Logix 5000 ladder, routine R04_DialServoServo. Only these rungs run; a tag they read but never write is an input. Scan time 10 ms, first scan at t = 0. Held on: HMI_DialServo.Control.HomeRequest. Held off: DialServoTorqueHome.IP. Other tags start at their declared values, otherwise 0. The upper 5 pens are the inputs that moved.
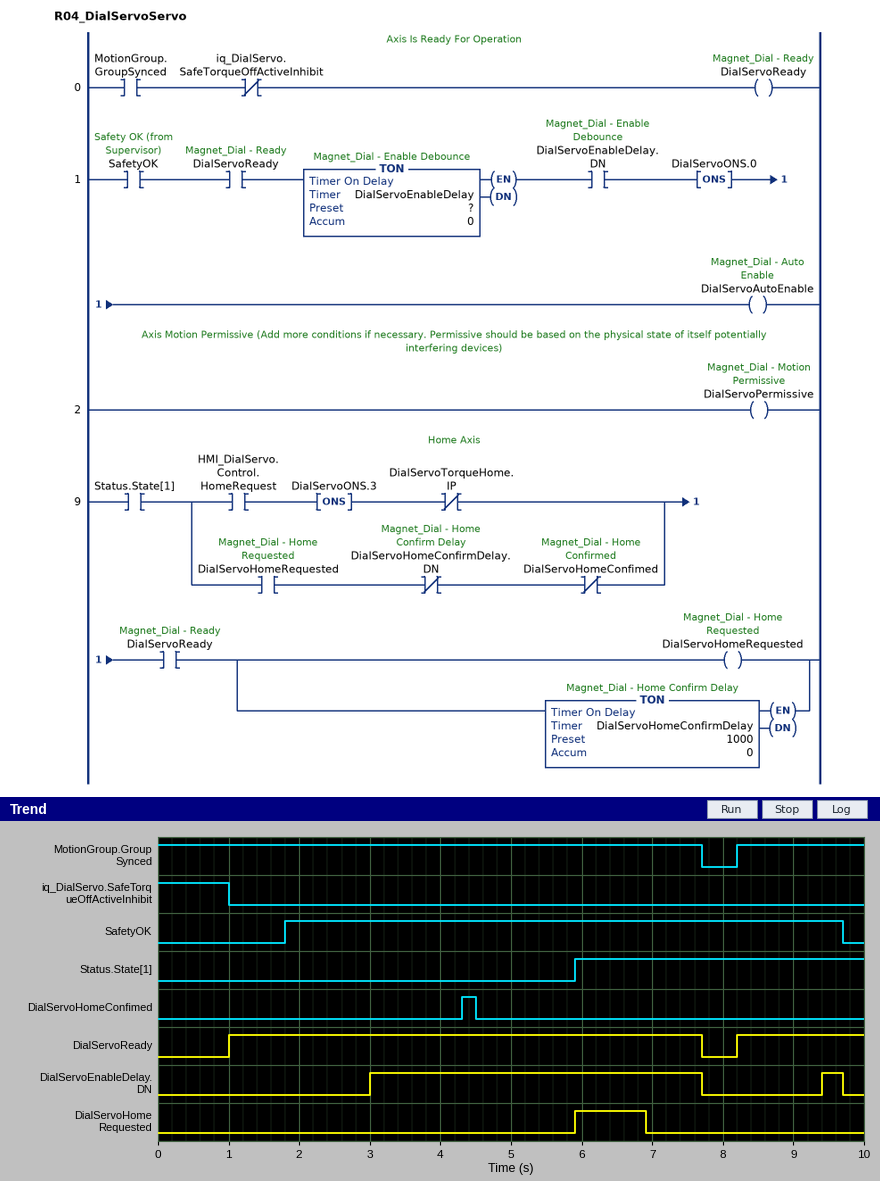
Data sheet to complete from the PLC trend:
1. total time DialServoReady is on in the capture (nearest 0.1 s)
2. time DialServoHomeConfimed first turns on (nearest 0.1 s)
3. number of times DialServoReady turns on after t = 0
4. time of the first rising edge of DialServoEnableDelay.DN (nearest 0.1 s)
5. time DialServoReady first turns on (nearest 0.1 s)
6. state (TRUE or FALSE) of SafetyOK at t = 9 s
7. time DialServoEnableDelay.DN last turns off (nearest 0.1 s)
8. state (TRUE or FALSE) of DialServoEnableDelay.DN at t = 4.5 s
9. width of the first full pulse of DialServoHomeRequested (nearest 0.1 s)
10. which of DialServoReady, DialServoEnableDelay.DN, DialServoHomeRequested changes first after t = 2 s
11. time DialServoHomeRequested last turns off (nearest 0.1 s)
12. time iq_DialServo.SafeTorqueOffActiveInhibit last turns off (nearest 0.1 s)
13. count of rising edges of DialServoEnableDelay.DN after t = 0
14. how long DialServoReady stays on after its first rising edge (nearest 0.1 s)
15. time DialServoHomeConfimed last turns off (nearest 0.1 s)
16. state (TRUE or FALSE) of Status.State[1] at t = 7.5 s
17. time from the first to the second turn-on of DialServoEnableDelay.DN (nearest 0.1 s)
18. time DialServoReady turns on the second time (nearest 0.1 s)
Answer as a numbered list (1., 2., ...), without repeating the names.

1. 8.5 s
2. 4.3 s
3. 2
4. 3.0 s
5. 1.0 s
6. TRUE
7. 9.7 s
8. TRUE
9. 1.0 s
10. DialServoEnableDelay.DN
11. 6.9 s
12. 1.0 s
13. 2
14. 6.7 s
15. 4.5 s
16. TRUE
17. 6.4 s
18. 8.2 s
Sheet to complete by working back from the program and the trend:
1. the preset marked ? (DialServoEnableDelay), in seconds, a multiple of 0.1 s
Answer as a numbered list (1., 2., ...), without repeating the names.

1. 1.2 s
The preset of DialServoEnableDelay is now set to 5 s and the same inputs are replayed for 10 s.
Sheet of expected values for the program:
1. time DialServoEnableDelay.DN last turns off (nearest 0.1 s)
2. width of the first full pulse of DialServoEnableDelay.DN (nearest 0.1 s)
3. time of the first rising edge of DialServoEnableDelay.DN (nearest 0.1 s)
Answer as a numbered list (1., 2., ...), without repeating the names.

1. 7.7 s
2. 0.9 s
3. 6.8 s
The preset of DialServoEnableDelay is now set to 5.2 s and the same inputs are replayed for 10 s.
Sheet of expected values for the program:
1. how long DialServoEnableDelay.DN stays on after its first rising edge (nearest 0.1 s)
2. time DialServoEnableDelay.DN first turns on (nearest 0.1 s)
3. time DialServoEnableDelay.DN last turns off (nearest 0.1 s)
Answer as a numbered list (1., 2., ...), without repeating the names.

1. 0.7 s
2. 7.0 s
3. 7.7 s
